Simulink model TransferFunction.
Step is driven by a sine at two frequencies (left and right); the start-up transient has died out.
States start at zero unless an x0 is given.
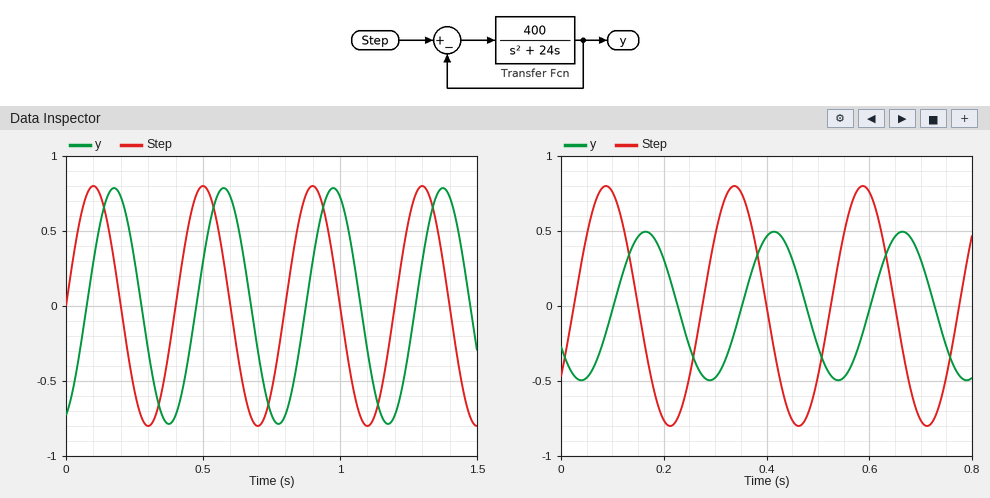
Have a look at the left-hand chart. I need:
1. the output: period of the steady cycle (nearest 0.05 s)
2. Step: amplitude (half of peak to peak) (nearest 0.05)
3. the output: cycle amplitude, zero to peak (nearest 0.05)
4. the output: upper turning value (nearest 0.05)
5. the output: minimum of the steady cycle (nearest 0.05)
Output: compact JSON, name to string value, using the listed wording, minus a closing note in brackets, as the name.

{"the output: period of the steady cycle": "0.40 s", "Step: amplitude (half of peak to peak)": "0.80", "the output: cycle amplitude, zero to peak": "0.80", "the output: upper turning value": "0.80", "the output: minimum of the steady cycle": "-0.80"}
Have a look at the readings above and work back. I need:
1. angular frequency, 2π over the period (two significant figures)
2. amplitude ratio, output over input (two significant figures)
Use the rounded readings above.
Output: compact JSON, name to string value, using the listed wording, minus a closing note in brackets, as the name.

{"angular frequency, 2π over the period": "16 rad/s", "amplitude ratio, output over input": "1.0"}
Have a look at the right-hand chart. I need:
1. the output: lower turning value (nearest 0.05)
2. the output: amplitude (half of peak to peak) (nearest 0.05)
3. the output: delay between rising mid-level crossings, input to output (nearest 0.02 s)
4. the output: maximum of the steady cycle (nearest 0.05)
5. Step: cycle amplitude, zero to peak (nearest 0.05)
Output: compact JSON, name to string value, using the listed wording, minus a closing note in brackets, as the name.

{"the output: lower turning value": "-0.50", "the output: amplitude (half of peak to peak)": "0.50", "the output: delay between rising mid-level crossings, input to output": "0.08 s", "the output: maximum of the steady cycle": "0.50", "Step: cycle amplitude, zero to peak": "0.80"}
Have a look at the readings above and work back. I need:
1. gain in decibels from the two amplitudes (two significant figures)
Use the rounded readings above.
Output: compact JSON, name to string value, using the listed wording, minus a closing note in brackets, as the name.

{"gain in decibels from the two amplitudes": "-4.1 dB"}
